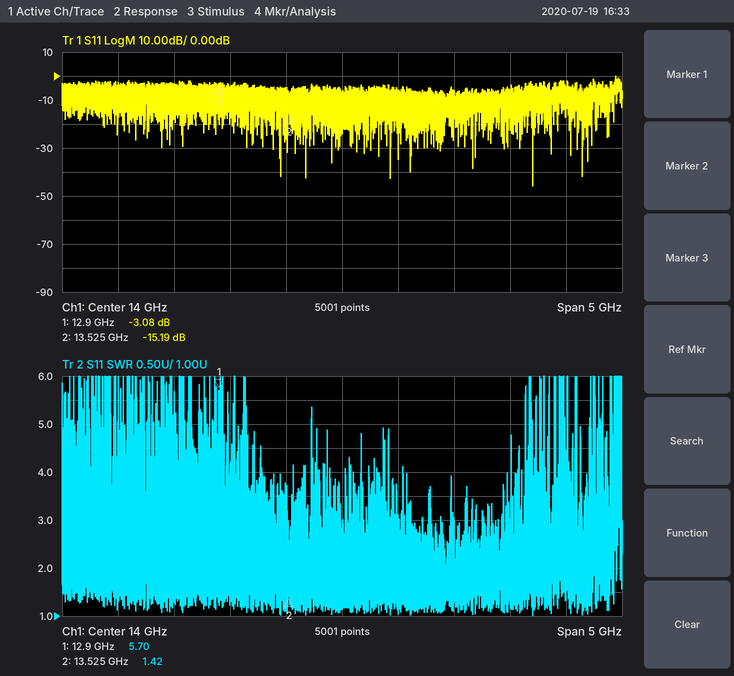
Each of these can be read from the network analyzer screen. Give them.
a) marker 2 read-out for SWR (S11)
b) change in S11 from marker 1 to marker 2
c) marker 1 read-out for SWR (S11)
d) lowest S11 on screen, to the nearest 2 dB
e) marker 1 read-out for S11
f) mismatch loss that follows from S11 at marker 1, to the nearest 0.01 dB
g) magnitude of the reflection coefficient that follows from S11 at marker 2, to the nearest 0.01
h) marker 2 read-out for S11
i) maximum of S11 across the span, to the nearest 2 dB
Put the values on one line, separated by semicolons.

1.42; -12.11 dB; 5.70; -46 dB; -3.08 dB; 2.94 dB; 0.17; -15.19 dB; 0 dB
